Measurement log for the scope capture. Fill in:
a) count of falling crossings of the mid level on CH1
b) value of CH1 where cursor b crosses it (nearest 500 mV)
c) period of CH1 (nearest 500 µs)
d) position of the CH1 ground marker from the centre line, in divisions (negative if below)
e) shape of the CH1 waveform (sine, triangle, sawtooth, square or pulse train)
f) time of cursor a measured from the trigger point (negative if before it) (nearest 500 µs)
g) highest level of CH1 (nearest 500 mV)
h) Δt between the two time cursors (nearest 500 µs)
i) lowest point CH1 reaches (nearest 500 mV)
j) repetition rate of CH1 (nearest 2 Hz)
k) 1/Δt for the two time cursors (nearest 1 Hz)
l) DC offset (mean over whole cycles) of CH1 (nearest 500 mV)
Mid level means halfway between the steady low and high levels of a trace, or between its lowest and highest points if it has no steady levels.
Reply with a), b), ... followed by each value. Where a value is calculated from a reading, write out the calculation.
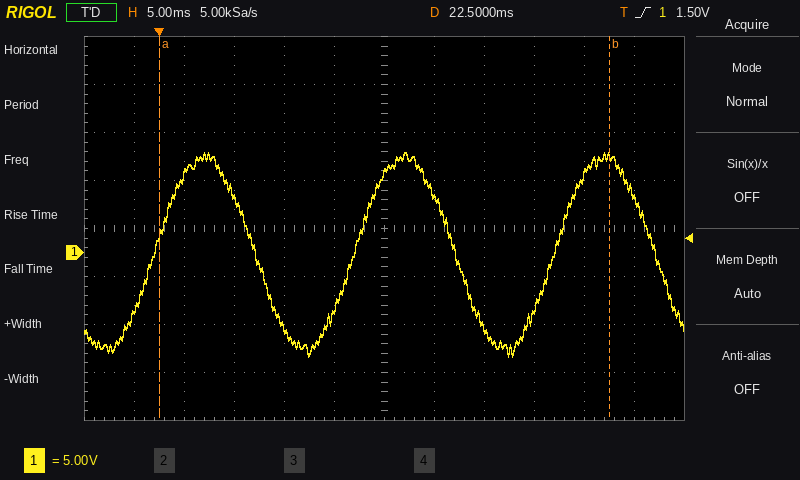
a) 3
b) 10.0 V
c) 20.0 ms
d) -0.5 div
e) sine
f) 0.0 ms
g) 10.5 V
h) 45.0 ms
i) -11.0 V
j) 1 / 20.0 ms ≈ 50 Hz
k) 1 / 45.0 ms ≈ 22 Hz
l) (10.5 V + (-11.0 V)) / 2 ≈ 0.0 V
